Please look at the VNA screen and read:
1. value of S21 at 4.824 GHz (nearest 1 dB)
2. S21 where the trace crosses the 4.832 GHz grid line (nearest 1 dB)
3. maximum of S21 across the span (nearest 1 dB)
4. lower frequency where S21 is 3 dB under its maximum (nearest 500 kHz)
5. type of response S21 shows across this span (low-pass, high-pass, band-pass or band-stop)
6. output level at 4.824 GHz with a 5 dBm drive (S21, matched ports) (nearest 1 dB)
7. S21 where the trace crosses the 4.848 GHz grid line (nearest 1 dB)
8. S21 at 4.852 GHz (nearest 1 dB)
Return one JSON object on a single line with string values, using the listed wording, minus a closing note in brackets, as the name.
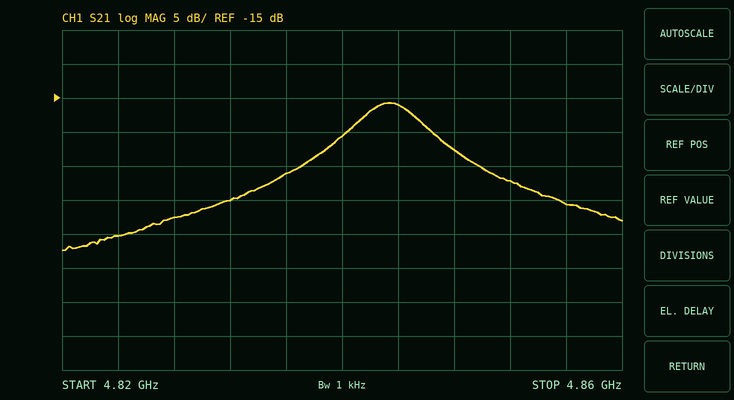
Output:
{"value of S21 at 4.824 GHz": "-35 dB", "S21 where the trace crosses the 4.832 GHz grid line": "-30 dB", "maximum of S21 across the span": "-16 dB", "lower frequency where S21 is 3 dB under its maximum": "4.8410 GHz", "type of response S21 shows across this span": "band-pass", "output level at 4.824 GHz with a 5 dBm drive (S21, matched ports)": "-30 dBm", "S21 where the trace crosses the 4.848 GHz grid line": "-23 dB", "S21 at 4.852 GHz": "-27 dB"}
